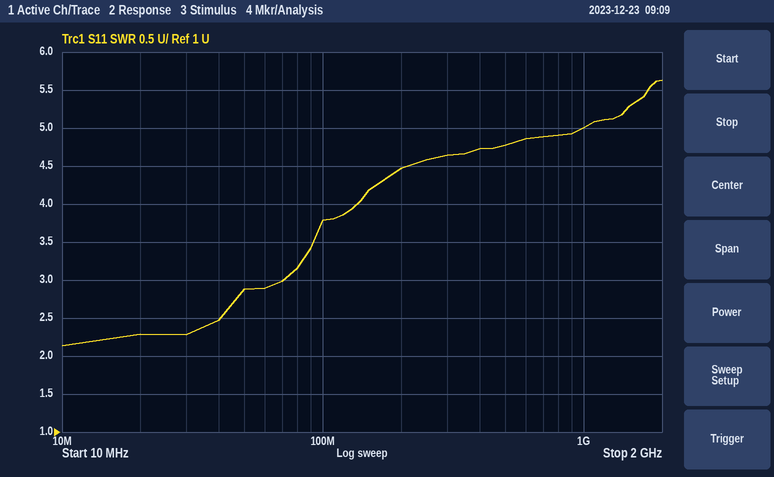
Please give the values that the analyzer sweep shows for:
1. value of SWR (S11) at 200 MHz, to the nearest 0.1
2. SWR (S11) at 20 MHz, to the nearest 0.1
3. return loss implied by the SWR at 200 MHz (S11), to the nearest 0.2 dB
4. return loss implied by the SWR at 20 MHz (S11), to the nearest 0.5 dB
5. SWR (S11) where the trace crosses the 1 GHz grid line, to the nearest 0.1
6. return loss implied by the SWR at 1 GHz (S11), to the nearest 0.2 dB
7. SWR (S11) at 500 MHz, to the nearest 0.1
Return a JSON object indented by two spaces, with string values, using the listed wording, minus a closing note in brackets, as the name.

{
  "value of SWR (S11) at 200 MHz, to the nearest 0.1": "4.5",
  "SWR (S11) at 20 MHz, to the nearest 0.1": "2.3",
  "return loss implied by the SWR at 200 MHz (S11), to the nearest 0.2 dB": "4.0 dB",
  "return loss implied by the SWR at 20 MHz (S11), to the nearest 0.5 dB": "8.0 dB",
  "SWR (S11) where the trace crosses the 1 GHz grid line, to the nearest 0.1": "5.0",
  "return loss implied by the SWR at 1 GHz (S11), to the nearest 0.2 dB": "3.6 dB",
  "SWR (S11) at 500 MHz, to the nearest 0.1": "4.8"
}
